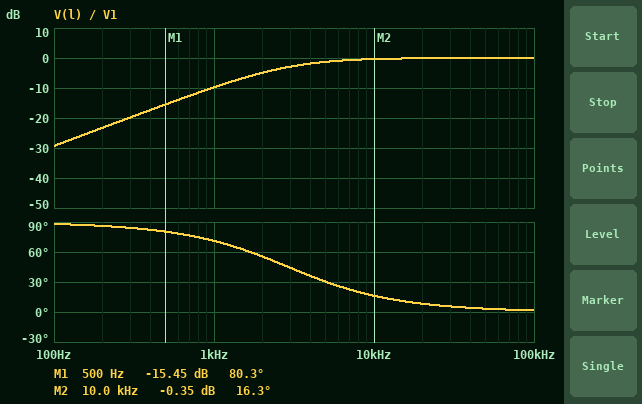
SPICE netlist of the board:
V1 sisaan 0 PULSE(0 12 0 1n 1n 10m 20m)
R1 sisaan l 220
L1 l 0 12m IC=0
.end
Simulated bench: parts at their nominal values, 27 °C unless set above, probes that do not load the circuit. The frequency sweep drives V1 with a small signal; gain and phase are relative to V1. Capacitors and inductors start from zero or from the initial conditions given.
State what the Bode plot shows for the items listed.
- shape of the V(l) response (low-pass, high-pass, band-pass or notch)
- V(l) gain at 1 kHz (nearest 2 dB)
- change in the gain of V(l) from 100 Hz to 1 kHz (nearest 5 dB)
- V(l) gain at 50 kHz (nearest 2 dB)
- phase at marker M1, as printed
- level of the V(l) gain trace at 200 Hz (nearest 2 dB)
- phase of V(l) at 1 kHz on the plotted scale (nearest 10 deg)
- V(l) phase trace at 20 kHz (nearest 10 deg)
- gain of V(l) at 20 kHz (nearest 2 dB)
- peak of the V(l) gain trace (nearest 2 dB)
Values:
high-pass
-10 dB
20 dB
0 dB
80.3 deg
-24 dB
70 deg
10 deg
0 dB
0 dB
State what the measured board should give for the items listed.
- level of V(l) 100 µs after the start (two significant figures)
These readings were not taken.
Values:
1.9 V
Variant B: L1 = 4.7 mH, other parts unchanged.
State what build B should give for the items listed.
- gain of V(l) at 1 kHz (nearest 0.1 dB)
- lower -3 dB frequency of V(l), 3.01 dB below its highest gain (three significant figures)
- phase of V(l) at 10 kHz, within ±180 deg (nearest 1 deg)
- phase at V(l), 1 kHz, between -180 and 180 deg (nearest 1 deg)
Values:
-17.5 dB
7.45 kHz
37 deg
82 deg
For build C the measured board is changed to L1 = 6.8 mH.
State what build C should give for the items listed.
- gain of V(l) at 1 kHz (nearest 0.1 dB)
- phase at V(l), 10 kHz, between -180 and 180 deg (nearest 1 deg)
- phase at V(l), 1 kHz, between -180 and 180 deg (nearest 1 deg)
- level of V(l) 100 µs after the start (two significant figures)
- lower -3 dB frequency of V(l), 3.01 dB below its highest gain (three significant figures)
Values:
-14.4 dB
27 deg
79 deg
470 mV
5.15 kHz
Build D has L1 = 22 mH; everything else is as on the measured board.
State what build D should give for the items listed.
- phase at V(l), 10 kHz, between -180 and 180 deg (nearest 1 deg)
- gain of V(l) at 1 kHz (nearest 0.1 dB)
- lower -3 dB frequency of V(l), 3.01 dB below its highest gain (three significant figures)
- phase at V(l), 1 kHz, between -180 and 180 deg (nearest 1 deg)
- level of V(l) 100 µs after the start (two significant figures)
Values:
9 deg
-5.5 dB
1.59 kHz
58 deg
4.4 V
